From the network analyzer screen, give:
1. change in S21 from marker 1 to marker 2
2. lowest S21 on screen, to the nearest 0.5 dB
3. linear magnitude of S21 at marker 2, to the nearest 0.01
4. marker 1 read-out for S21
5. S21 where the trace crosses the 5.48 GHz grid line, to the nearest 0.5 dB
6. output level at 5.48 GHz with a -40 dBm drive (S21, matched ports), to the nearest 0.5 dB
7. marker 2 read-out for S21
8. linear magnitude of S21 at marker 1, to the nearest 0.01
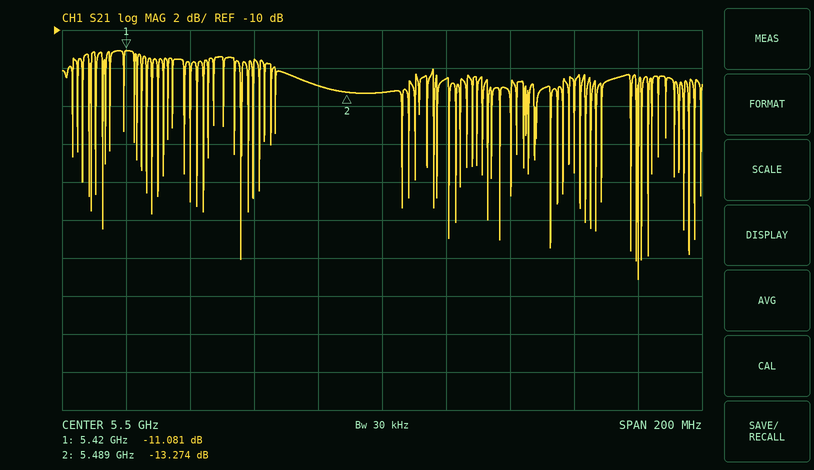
-2.193 dB
-23.0 dB
0.22
-11.081 dB
-13.0 dB
-53.0 dBm
-13.274 dB
0.28
